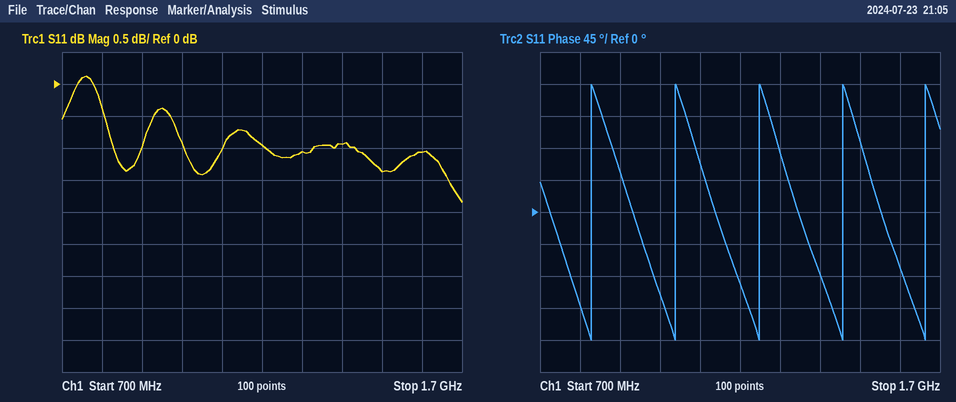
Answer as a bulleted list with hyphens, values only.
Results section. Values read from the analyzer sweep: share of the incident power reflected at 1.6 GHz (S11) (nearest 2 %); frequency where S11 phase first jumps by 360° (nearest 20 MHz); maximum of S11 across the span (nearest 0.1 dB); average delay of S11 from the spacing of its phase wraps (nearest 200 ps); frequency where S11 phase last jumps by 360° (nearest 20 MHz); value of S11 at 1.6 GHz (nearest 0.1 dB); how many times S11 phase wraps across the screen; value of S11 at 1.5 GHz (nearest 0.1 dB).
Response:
- 78 %
- 820 MHz
- 0.1 dB
- 4.8 ns
- 1.66 GHz
- -1.1 dB
- 5
- -1.4 dB
